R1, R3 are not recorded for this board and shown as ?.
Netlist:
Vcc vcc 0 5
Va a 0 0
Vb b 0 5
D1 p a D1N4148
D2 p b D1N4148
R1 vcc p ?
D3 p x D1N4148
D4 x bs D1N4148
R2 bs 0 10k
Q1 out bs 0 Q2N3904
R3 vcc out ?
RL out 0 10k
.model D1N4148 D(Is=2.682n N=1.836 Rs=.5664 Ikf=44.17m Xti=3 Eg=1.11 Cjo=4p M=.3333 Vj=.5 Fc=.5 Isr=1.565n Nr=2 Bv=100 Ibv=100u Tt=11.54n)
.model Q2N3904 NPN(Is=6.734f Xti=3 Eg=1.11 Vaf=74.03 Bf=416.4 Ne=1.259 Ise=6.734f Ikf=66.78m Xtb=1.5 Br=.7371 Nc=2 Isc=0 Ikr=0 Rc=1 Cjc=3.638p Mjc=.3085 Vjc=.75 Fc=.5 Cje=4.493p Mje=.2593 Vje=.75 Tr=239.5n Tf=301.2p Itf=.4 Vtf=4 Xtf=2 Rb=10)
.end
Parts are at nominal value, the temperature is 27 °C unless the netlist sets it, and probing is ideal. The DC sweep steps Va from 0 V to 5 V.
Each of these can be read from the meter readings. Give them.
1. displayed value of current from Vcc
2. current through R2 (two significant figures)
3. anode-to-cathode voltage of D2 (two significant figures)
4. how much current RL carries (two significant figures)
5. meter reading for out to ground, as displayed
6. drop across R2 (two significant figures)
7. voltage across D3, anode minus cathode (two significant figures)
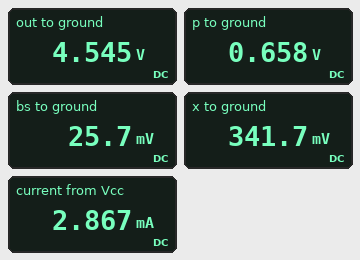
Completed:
2.867 mA
2.6 µA
-4.3 V
450 µA
4.545 V
26 mV
320 mV
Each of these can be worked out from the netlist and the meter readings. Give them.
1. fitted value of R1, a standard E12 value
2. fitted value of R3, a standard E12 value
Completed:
1.8 kΩ
1 kΩ
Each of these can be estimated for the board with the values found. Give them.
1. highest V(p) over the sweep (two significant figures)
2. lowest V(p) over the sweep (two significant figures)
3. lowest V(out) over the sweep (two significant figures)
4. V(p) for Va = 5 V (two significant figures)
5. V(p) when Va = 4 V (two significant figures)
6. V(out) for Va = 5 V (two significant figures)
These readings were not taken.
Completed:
2.0 V
660 mV
57 mV
2.0 V
2.0 V
57 mV
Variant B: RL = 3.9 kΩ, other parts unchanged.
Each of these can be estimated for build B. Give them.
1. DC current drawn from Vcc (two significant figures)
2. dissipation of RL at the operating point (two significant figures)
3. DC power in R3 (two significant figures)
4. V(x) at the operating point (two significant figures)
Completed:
3.4 mA
4.1 mW
1.0 mW
340 mV
